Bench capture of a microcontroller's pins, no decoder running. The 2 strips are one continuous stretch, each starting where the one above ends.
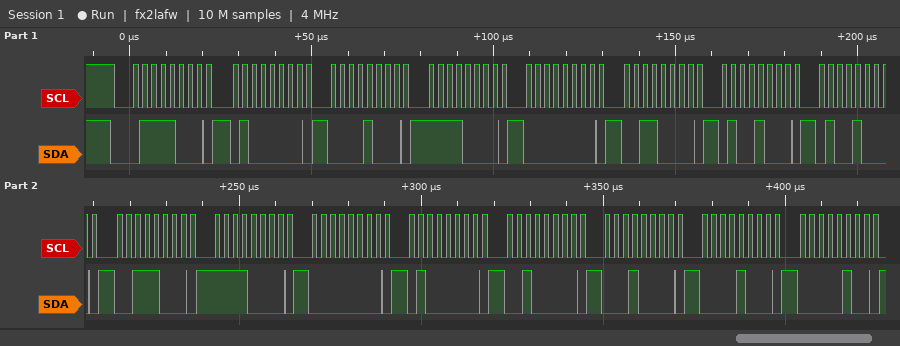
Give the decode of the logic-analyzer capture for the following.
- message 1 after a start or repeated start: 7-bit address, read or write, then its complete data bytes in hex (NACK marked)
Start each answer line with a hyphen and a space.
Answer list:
- 0x3C write: 40 08 F0 00 30 48 48 38 F0 00 40 20 10 08 04
